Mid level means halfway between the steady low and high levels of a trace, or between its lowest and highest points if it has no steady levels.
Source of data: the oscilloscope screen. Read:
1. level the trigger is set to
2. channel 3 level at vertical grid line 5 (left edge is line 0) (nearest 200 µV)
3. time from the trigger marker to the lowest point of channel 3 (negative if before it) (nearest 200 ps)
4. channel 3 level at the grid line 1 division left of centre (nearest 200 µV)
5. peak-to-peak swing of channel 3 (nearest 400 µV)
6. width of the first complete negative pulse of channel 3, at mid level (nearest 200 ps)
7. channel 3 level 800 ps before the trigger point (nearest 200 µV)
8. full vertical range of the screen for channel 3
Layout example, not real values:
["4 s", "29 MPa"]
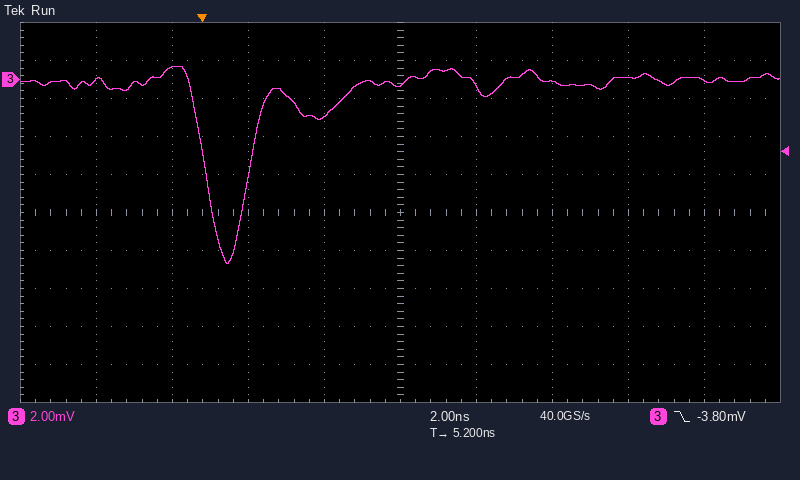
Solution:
["-3.80 mV", "-200 µV", "+600 ps", "-2.0 mV", "10.4 mV", "1.2 ns", "600 µV", "20 mV"]
